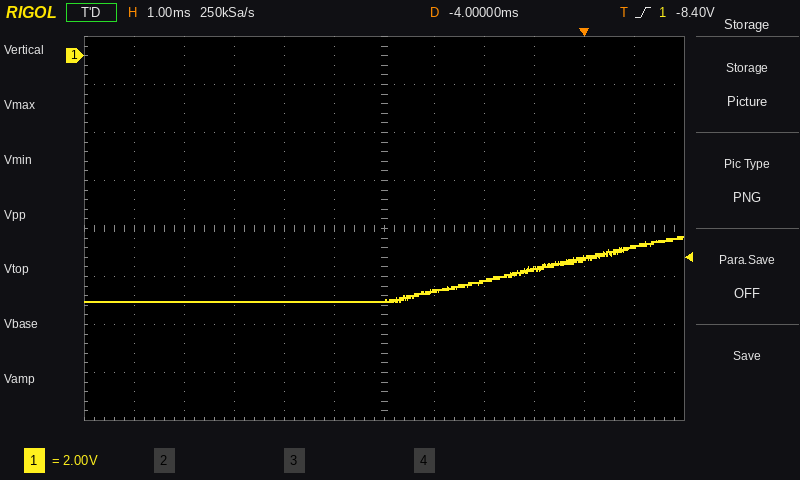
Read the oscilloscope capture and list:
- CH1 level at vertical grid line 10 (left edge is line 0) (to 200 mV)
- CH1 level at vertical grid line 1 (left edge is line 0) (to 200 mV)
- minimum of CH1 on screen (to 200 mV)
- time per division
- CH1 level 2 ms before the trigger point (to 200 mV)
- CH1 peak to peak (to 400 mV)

-8.4 V
-10.2 V
-10.2 V
1 ms
-9.4 V
2.8 V
